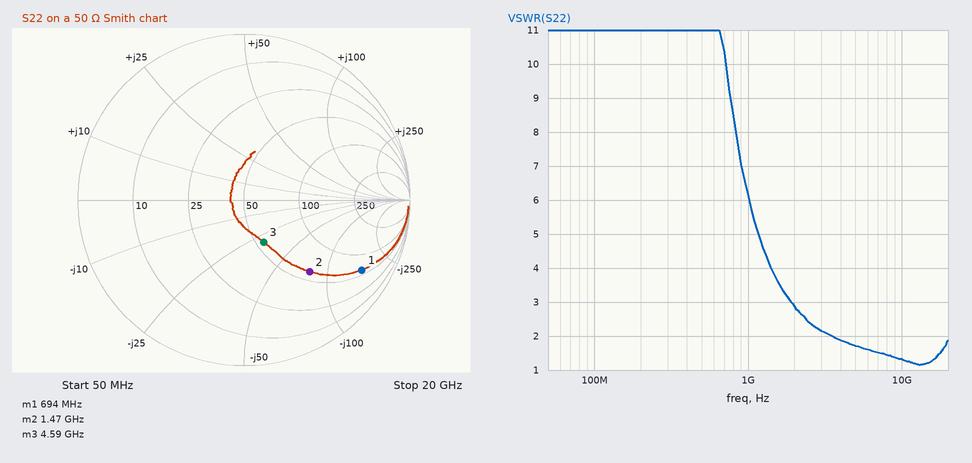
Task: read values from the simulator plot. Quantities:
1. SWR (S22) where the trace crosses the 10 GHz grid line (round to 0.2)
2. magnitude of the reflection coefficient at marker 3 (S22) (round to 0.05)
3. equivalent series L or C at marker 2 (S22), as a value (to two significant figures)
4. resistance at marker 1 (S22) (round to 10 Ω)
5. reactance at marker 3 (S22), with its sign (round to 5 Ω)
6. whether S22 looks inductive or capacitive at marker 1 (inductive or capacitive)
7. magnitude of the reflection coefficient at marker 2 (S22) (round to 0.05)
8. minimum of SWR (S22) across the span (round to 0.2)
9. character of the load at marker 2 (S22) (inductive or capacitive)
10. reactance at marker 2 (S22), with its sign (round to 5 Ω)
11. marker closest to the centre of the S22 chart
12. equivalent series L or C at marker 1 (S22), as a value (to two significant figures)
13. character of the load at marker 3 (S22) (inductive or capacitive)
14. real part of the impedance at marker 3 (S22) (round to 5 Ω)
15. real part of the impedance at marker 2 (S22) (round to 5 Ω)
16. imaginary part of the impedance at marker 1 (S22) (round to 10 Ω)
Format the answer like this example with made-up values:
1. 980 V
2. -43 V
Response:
1. 1.4
2. 0.30
3. 1.4 pF
4. 60 Ω
5. -30 Ω
6. capacitive
7. 0.60
8. 1.2
9. capacitive
10. -80 Ω
11. marker 3
12. 1.4 pF
13. capacitive
14. 55 Ω
15. 60 Ω
16. -160 Ω
